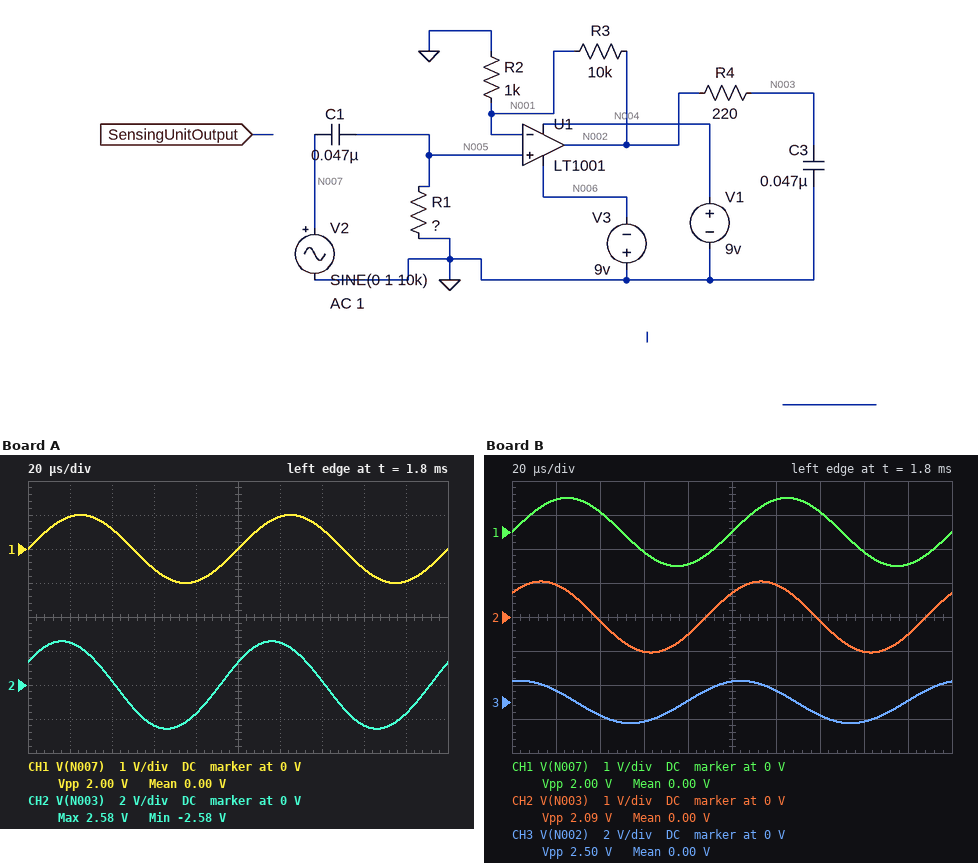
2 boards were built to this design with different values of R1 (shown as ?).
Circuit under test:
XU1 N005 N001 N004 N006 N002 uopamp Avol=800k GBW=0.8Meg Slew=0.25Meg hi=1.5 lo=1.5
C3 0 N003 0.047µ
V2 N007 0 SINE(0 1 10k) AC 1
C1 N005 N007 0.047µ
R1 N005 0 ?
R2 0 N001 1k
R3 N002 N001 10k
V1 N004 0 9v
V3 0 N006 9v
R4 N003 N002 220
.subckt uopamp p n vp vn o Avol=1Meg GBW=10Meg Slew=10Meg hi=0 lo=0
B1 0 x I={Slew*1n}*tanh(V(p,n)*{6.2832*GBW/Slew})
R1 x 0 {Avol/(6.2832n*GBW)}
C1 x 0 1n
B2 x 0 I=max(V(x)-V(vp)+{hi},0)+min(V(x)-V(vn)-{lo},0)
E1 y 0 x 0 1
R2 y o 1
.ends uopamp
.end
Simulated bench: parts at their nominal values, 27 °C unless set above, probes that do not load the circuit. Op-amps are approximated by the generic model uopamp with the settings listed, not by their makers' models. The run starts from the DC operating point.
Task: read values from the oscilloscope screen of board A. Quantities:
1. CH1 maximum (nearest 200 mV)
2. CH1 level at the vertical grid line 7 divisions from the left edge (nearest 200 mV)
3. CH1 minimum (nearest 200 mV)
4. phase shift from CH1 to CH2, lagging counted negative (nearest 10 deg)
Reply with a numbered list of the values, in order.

1. 1.0 V
2. 600 mV
3. -1.0 V
4. 30 deg
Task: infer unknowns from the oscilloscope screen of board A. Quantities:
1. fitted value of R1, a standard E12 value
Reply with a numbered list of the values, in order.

1. 100 Ω
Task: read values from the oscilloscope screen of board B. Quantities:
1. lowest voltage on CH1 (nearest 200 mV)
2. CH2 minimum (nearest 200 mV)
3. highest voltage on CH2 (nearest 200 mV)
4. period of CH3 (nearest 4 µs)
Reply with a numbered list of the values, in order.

1. -1.0 V
2. -1.0 V
3. 1.0 V
4. 100 µs
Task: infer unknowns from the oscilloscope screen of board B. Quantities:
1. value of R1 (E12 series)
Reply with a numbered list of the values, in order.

1. 39 Ω
